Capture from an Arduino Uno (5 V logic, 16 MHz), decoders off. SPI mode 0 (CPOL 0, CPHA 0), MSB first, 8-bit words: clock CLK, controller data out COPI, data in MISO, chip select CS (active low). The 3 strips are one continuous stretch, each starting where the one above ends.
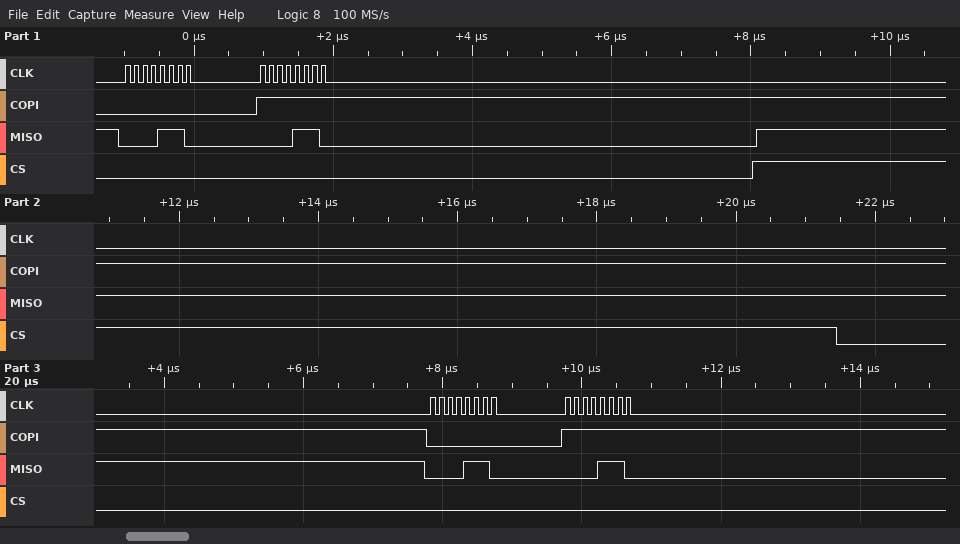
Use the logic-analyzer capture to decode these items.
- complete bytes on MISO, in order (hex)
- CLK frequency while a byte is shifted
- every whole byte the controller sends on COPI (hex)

0x0E 0x0E 0x0E 0x0E
8 MHz
0x00 0xFF 0x00 0xFF
